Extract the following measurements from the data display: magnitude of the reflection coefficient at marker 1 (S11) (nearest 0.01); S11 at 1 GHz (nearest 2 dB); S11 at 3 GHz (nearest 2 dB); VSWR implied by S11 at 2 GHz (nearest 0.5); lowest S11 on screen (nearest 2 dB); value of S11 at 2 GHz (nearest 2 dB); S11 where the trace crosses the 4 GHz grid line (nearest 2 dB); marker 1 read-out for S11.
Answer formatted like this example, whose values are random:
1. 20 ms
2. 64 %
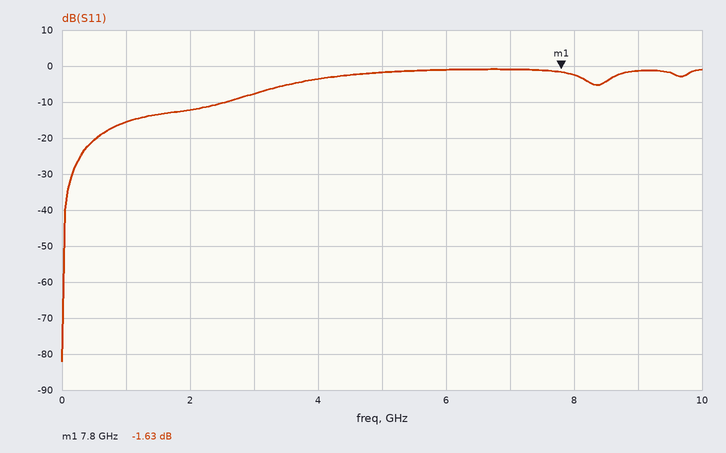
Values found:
1. 0.83
2. -16 dB
3. -8 dB
4. 1.5
5. -82 dB
6. -12 dB
7. -4 dB
8. -1.63 dB
